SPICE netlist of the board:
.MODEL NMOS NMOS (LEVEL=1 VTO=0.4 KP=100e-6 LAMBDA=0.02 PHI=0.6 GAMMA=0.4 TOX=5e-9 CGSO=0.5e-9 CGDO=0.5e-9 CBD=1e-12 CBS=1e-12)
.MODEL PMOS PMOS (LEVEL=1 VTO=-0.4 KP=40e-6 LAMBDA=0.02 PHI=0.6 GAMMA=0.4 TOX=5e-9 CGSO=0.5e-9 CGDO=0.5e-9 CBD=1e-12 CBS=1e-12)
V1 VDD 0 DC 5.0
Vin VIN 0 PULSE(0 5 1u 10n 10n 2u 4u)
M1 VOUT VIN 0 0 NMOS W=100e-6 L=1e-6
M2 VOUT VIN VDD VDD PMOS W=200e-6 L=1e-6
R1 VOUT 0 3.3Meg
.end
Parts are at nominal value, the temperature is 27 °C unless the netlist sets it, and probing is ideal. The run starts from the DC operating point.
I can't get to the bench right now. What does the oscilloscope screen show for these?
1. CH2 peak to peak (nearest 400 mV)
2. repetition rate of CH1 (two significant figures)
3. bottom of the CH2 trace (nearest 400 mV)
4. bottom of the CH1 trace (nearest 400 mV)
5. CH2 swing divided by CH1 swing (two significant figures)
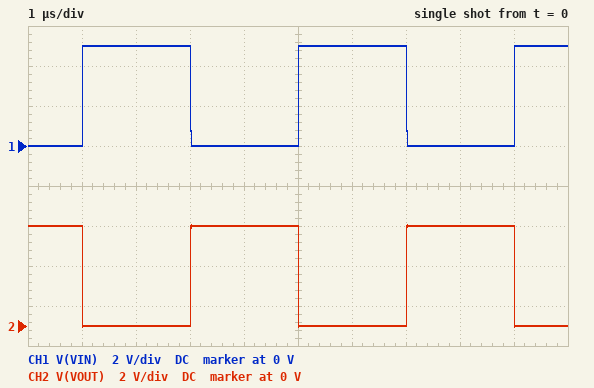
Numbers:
5.2 V
250 kHz
0 V
0 V
1.0
